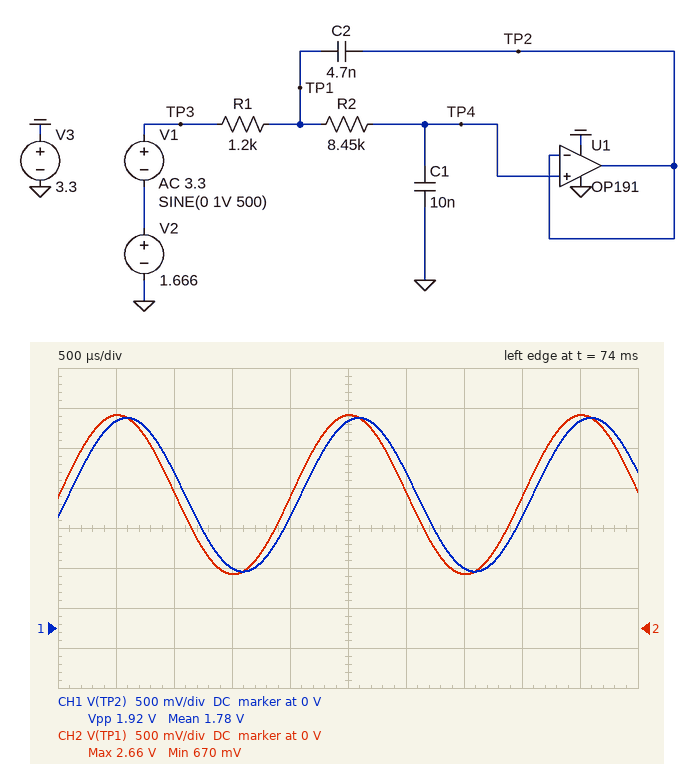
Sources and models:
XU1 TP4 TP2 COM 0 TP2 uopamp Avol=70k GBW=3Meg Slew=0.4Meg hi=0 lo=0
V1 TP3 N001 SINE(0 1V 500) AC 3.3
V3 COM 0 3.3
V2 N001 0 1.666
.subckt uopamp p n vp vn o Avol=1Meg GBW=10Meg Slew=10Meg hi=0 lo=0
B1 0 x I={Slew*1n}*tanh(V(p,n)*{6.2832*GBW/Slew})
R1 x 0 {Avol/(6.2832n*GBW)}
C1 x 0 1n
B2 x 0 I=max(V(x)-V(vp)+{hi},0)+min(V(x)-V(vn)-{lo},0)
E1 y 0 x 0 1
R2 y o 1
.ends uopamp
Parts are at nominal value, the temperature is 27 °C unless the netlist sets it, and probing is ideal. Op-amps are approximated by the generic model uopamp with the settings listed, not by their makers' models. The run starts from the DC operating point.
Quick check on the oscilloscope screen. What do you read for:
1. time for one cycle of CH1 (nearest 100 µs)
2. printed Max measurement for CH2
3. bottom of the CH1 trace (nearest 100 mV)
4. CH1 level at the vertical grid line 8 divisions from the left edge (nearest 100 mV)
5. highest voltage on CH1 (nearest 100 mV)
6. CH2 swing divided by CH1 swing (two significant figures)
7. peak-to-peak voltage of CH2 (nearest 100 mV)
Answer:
2.0 ms
2.66 V
700 mV
1.4 V
2.6 V
1.0
2.0 V
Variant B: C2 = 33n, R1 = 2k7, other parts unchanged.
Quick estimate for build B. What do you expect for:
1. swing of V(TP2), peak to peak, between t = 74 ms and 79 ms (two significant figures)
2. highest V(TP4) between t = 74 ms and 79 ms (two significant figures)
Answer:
2.0 V
2.7 V
